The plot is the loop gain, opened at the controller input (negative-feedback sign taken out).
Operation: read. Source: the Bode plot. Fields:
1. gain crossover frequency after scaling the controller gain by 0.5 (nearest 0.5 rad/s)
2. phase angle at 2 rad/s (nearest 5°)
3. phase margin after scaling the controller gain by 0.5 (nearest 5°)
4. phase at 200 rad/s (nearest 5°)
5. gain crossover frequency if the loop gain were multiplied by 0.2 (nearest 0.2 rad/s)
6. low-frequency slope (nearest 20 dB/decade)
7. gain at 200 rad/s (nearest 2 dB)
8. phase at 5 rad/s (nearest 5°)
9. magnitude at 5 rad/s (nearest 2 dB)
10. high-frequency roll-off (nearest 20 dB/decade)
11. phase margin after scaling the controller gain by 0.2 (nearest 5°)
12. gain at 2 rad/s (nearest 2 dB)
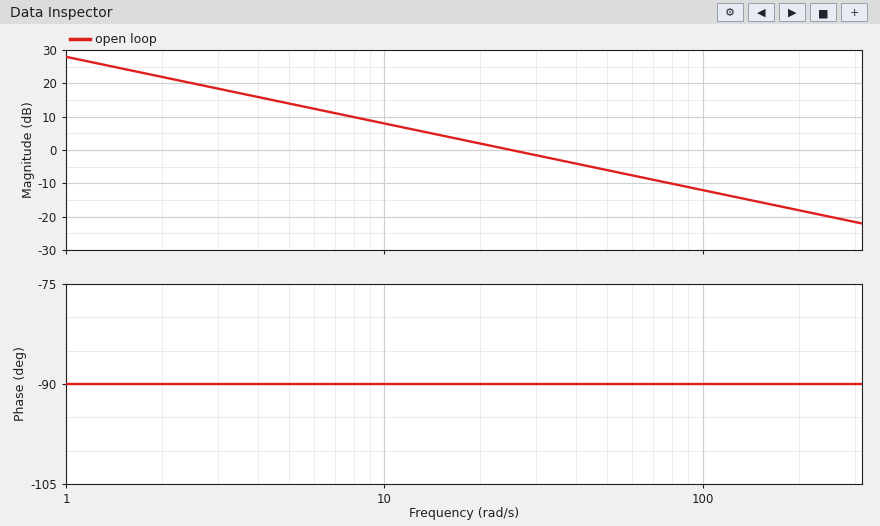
12.5 rad/s
-90°
90°
-90°
5.0 rad/s
-20 dB/decade
-18 dB
-90°
14 dB
-20 dB/decade
90°
22 dB
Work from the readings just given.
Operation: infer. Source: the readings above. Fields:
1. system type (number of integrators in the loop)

1
